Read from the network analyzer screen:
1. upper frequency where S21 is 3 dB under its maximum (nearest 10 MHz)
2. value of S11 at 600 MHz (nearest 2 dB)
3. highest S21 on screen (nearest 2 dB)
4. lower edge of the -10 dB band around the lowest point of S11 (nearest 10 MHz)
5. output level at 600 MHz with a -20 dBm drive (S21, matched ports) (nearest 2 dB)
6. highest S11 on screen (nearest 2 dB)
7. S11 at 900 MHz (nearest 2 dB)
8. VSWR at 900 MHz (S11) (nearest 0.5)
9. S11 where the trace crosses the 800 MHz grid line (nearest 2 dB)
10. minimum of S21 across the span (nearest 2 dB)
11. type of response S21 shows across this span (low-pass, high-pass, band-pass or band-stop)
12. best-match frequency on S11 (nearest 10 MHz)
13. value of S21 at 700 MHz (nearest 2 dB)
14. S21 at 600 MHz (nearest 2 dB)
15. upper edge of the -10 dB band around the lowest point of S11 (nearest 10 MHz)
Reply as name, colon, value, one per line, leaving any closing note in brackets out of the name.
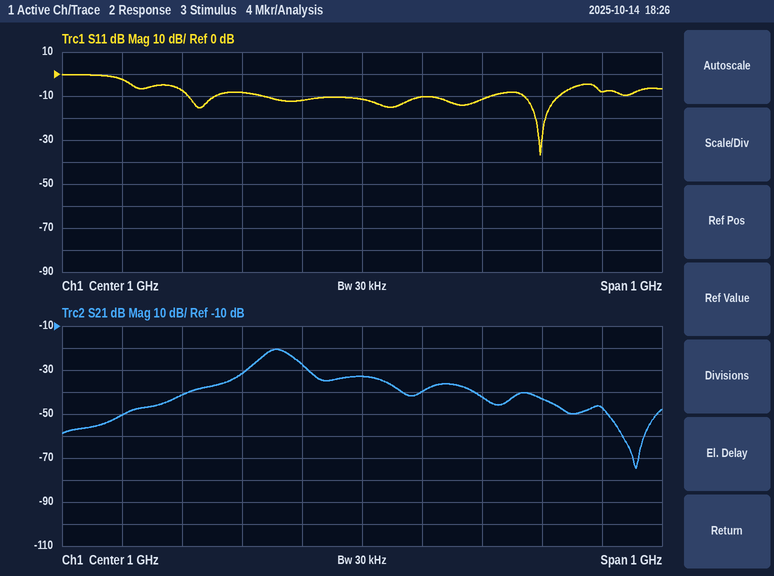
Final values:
upper frequency where S21 is 3 dB under its maximum: 880 MHz
value of S11 at 600 MHz: -2 dB
highest S21 on screen: -20 dB
lower edge of the -10 dB band around the lowest point of S11: 1.27 GHz
output level at 600 MHz with a -20 dBm drive (S21, matched ports): -70 dBm
highest S11 on screen: 0 dB
S11 at 900 MHz: -12 dB
VSWR at 900 MHz (S11): 1.5
S11 where the trace crosses the 800 MHz grid line: -8 dB
minimum of S21 across the span: -74 dB
type of response S21 shows across this span: band-pass
best-match frequency on S11: 1.30 GHz
value of S21 at 700 MHz: -42 dB
S21 at 600 MHz: -50 dB
upper edge of the -10 dB band around the lowest point of S11: 1.33 GHz
